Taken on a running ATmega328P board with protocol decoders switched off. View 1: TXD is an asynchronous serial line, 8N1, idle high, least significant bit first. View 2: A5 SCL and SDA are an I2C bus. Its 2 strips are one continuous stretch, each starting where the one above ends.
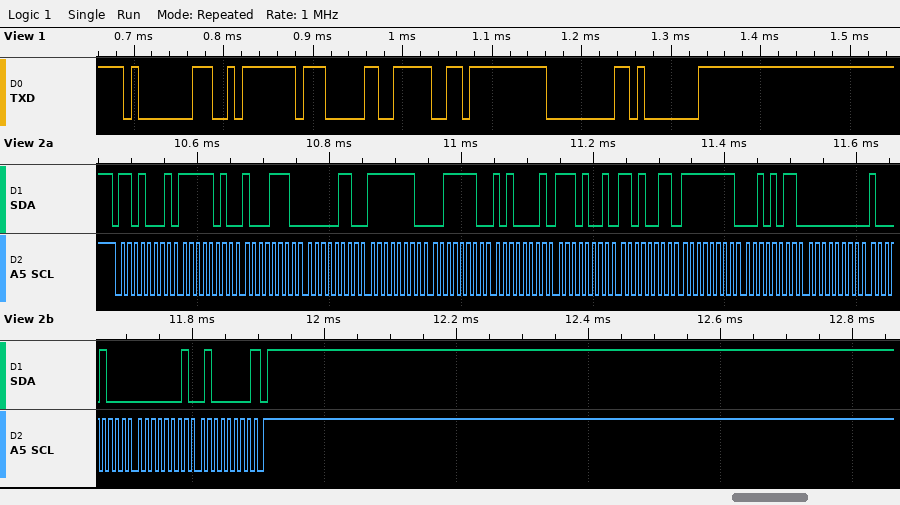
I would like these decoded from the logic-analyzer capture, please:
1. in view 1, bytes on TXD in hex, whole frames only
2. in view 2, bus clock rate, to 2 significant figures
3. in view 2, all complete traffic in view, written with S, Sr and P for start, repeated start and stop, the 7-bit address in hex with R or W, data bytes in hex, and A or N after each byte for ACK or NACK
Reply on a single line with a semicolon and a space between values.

01 FA 07 3E FF 00 01; 100 kHz; S 68R A FA A 8E A 06 A FE A 3E A A1 A E9 A D3 A FF A 2B A 00 A 88 A 01 A 40 N P
